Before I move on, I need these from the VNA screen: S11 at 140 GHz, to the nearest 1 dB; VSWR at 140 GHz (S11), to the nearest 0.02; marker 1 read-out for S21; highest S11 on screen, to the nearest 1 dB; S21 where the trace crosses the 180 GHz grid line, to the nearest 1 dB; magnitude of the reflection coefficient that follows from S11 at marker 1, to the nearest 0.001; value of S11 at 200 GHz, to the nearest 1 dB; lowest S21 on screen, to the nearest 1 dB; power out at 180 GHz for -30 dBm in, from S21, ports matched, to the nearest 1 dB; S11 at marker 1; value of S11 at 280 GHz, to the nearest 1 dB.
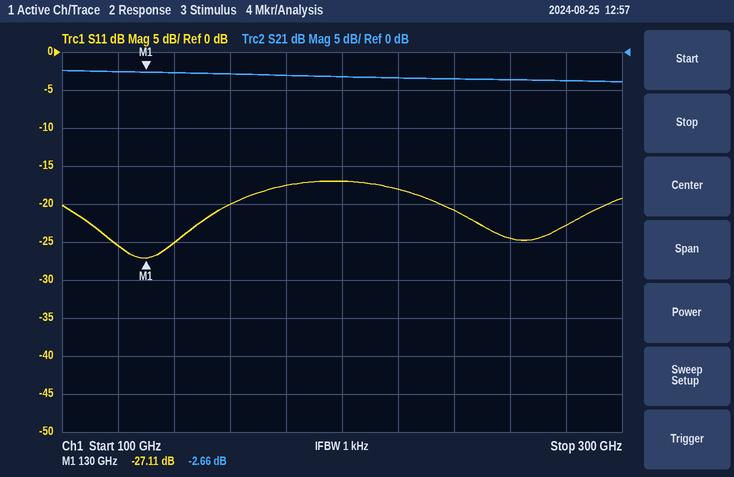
-25 dB
1.12
-2.66 dB
-17 dB
-3 dB
0.044
-17 dB
-4 dB
-33 dBm
-27.11 dB
-23 dB
